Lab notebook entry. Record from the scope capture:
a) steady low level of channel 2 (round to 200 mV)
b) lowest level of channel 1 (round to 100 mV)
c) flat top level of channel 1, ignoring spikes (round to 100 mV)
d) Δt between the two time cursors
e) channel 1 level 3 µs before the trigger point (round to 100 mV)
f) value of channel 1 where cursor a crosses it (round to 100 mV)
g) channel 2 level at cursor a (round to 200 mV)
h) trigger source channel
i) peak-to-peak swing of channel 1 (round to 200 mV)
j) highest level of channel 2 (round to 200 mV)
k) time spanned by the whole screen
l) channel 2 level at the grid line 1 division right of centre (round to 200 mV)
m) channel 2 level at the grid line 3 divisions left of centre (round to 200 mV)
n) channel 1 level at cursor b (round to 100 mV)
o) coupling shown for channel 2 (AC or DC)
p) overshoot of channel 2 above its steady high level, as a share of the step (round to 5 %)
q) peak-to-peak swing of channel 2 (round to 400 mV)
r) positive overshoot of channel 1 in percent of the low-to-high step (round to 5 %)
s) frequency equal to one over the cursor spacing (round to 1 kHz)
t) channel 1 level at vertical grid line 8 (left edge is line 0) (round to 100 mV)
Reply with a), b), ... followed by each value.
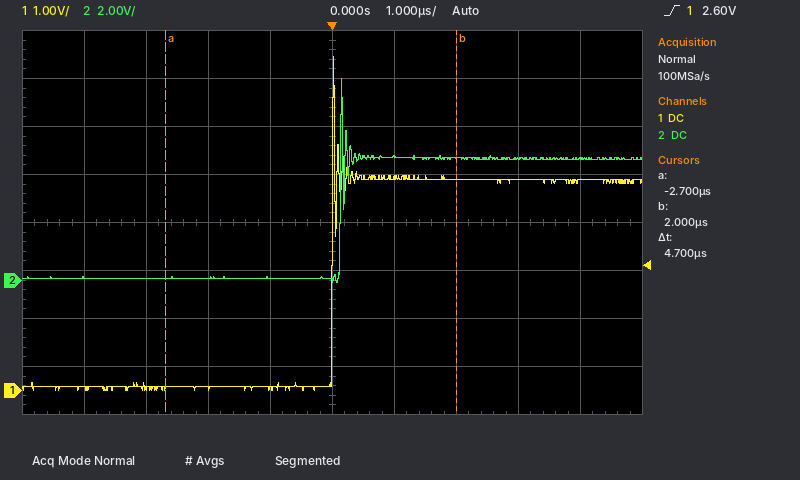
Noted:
a) 0.0 V
b) 0.0 V
c) 4.4 V
d) 4.7 µs
e) 100 mV
f) 0.0 V
g) 0.0 V
h) channel 1
i) 7.0 V
j) 8.4 V
k) 10 µs
l) 5.2 V
m) 0.0 V
n) 4.4 V
o) DC
p) 65 %
q) 8.4 V
r) 60 %
s) 213 kHz
t) 4.4 V
